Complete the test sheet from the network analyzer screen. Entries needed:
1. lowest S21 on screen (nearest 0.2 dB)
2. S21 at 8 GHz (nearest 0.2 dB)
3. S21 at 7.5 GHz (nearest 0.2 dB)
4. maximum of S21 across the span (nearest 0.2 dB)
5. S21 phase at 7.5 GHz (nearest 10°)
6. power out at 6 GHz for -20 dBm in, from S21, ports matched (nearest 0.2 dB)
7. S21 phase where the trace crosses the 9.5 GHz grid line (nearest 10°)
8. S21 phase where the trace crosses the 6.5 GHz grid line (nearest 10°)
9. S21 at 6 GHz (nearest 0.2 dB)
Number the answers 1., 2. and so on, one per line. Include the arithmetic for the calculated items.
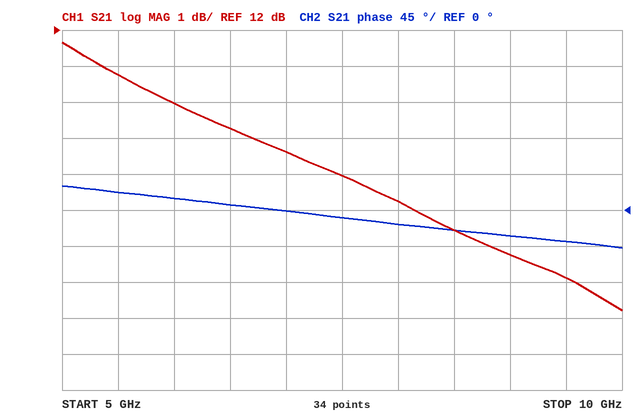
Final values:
1. 4.2 dB
2. 7.2 dB
3. 8.0 dB
4. 11.6 dB
5. -10°
6. -20 dBm + (10.0 dB) = -10.0 dBm
7. -40°
8. 10°
9. 10.0 dB
